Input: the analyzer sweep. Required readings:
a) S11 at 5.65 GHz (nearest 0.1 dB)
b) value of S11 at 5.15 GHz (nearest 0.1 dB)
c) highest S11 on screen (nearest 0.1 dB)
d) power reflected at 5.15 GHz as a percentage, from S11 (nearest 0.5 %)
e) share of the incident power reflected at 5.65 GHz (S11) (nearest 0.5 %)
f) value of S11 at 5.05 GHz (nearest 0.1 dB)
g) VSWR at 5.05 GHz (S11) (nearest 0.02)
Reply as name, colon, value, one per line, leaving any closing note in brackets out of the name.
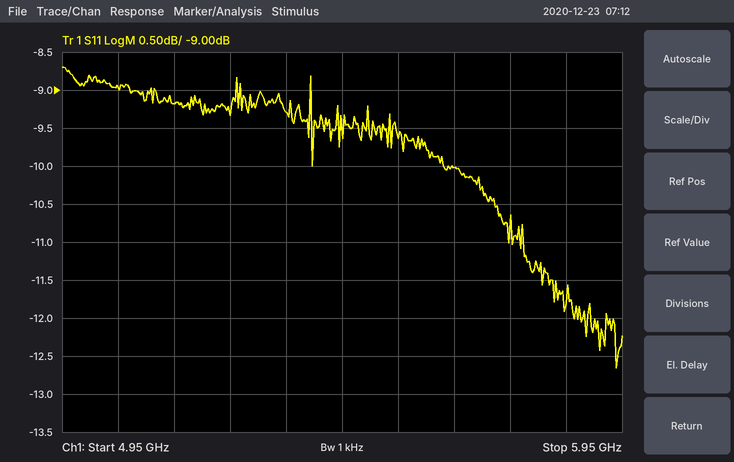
S11 at 5.65 GHz: -10.0 dB
value of S11 at 5.15 GHz: -9.2 dB
highest S11 on screen: -8.7 dB
power reflected at 5.15 GHz as a percentage, from S11: 12.0 %
share of the incident power reflected at 5.65 GHz (S11): 10.0 %
value of S11 at 5.05 GHz: -9.0 dB
VSWR at 5.05 GHz (S11): 2.10
